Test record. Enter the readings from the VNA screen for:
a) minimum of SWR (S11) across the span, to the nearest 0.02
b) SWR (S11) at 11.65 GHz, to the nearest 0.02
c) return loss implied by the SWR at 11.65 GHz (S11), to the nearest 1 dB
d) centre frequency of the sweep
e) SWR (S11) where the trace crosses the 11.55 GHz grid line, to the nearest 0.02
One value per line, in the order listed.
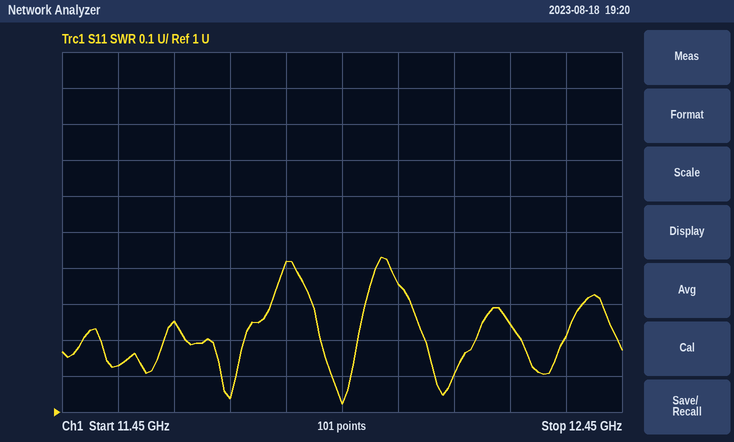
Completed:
1.02
1.26
19 dB
11.95 GHz
1.12
